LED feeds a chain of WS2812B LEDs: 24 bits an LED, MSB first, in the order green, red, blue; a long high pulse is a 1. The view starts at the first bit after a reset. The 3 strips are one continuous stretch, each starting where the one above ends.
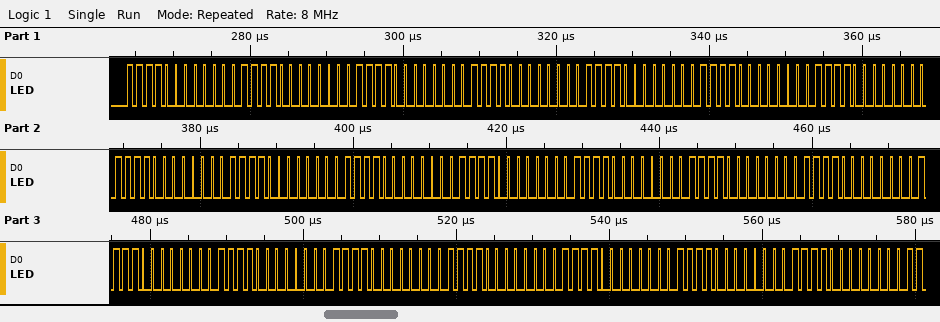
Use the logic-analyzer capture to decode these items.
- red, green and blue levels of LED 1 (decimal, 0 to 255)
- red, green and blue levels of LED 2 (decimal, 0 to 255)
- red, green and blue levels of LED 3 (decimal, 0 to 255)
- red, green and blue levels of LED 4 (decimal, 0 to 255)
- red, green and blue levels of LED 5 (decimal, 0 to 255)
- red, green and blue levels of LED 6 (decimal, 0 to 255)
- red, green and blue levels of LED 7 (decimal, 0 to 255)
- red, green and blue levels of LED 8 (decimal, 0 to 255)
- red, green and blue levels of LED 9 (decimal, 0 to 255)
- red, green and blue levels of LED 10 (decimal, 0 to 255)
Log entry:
15, 240, 0
15, 240, 0
15, 240, 0
15, 240, 0
15, 240, 0
15, 240, 0
15, 240, 0
15, 240, 0
15, 240, 0
15, 240, 0
